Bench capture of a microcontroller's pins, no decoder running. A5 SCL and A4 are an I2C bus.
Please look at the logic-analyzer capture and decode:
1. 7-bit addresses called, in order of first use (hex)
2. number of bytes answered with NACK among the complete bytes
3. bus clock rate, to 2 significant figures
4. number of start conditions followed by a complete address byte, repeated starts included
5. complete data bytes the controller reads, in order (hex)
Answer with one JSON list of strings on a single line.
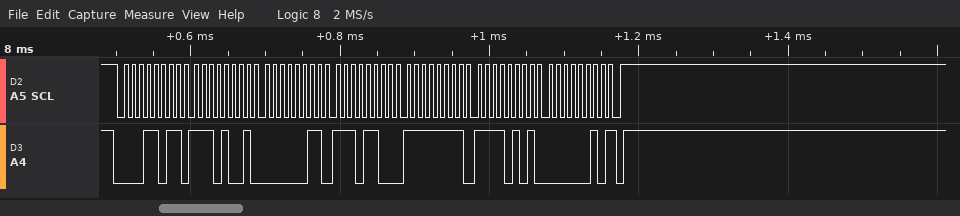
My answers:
["0x0D", "1", "100 kHz", "1", "E9 03 EC FF F5 02"]
